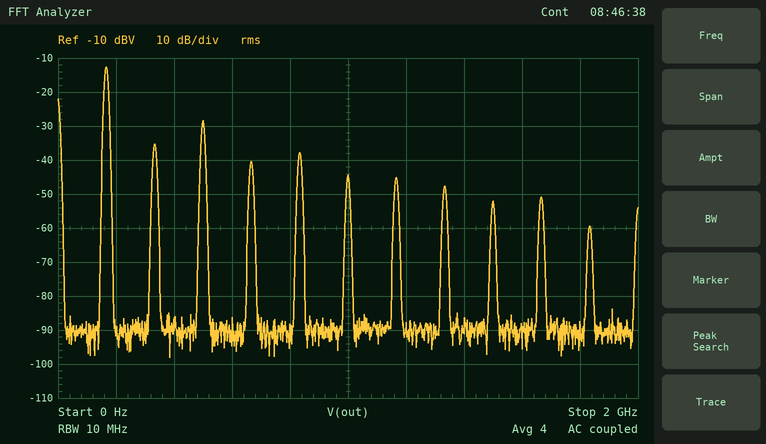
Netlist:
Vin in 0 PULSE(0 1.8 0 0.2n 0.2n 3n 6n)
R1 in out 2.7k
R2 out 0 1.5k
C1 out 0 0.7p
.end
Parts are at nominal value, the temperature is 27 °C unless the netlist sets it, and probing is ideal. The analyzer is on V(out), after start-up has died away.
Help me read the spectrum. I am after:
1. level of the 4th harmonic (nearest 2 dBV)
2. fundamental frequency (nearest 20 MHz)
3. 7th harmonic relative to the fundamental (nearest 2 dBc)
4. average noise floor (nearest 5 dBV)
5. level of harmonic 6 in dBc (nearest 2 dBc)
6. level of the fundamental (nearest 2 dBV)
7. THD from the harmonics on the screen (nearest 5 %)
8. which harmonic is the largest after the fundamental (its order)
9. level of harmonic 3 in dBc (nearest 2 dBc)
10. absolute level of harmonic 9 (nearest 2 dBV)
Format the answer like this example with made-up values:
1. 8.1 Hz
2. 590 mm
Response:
1. -40 dBV
2. 160 MHz
3. -32 dBc
4. -90 dBV
5. -32 dBc
6. -12 dBV
7. 20 %
8. 3
9. -16 dBc
10. -52 dBV
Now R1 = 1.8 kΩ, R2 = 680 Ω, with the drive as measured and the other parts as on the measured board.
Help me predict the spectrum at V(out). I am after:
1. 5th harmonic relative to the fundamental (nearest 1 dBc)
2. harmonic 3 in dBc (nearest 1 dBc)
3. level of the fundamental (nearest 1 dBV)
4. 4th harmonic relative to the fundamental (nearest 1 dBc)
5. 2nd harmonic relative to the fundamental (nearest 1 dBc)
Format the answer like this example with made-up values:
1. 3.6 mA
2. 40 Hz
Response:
1. -21 dBc
2. -13 dBc
3. -14 dBV
4. -24 dBc
5. -21 dBc
